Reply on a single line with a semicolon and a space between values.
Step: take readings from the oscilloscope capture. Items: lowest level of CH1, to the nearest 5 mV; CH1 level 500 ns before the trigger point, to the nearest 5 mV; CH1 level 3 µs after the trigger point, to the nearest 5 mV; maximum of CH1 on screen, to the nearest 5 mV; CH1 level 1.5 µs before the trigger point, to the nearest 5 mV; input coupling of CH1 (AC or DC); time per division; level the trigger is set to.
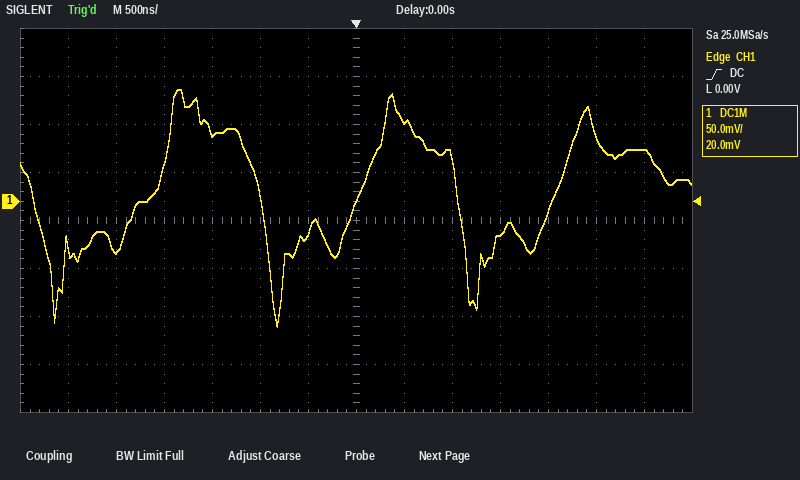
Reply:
-130 mV; -35 mV; 55 mV; 115 mV; 70 mV; DC; 500 ns; 0.00 V
